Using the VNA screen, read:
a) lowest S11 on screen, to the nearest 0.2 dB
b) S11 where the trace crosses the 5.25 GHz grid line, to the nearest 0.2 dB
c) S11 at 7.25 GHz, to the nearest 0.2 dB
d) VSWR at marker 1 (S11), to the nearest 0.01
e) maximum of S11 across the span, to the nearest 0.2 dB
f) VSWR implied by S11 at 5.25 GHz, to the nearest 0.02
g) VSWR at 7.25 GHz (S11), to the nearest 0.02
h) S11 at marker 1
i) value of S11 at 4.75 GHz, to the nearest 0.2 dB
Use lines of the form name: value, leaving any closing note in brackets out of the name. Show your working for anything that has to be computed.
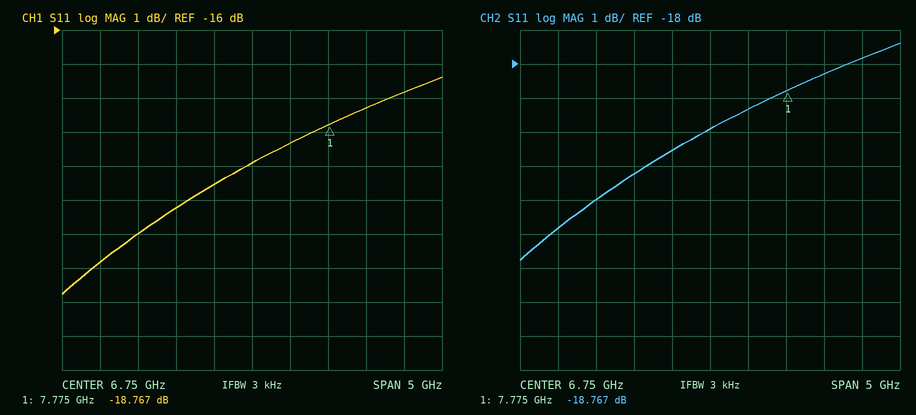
lowest S11 on screen, to the nearest 0.2 dB: -23.8 dB
S11 where the trace crosses the 5.25 GHz grid line, to the nearest 0.2 dB: -22.0 dB
S11 at 7.25 GHz, to the nearest 0.2 dB: -19.4 dB
VSWR at marker 1 (S11), to the nearest 0.01: (1 + 0.1153)/(1 − 0.1153) ≈ 1.26
maximum of S11 across the span, to the nearest 0.2 dB: -17.4 dB
VSWR implied by S11 at 5.25 GHz, to the nearest 0.02: |Γ| = 10^(-22/20) = 0.0794; VSWR = (1 + 0.0794)/(1 − 0.0794) ≈ 1.17, so 1.18 to the nearest 0.02
VSWR at 7.25 GHz (S11), to the nearest 0.02: |Γ| = 10^(-19.4/20) = 0.1072; VSWR = (1 + 0.1072)/(1 − 0.1072) ≈ 1.24
S11 at marker 1: -18.767 dB
value of S11 at 4.75 GHz, to the nearest 0.2 dB: -22.8 dB
